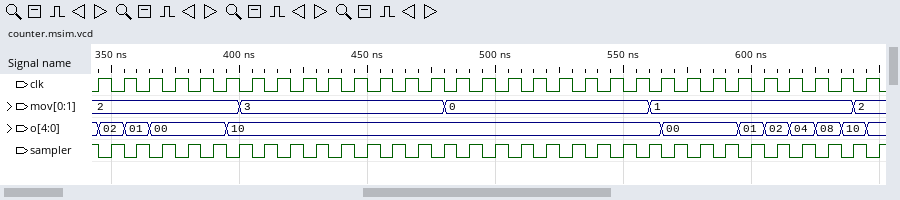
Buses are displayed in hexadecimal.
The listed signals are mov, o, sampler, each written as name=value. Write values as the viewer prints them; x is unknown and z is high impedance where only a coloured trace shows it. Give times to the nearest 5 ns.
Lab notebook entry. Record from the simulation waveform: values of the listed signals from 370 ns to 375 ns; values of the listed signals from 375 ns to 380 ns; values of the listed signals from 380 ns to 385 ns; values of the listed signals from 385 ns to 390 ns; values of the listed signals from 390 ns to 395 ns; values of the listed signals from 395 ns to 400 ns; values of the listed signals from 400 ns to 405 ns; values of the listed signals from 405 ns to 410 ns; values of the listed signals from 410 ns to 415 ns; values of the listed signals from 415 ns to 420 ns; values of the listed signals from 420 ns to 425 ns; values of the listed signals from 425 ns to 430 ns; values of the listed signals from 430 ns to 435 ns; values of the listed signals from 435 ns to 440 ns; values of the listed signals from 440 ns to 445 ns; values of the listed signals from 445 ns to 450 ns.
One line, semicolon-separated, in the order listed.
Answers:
mov=2, o=00, sampler=1; mov=2, o=00, sampler=0; mov=2, o=00, sampler=1; mov=2, o=00, sampler=0; mov=2, o=00, sampler=1; mov=2, o=10, sampler=0; mov=3, o=10, sampler=1; mov=3, o=10, sampler=0; mov=3, o=10, sampler=1; mov=3, o=10, sampler=0; mov=3, o=10, sampler=1; mov=3, o=10, sampler=0; mov=3, o=10, sampler=1; mov=3, o=10, sampler=0; mov=3, o=10, sampler=1; mov=3, o=10, sampler=0
